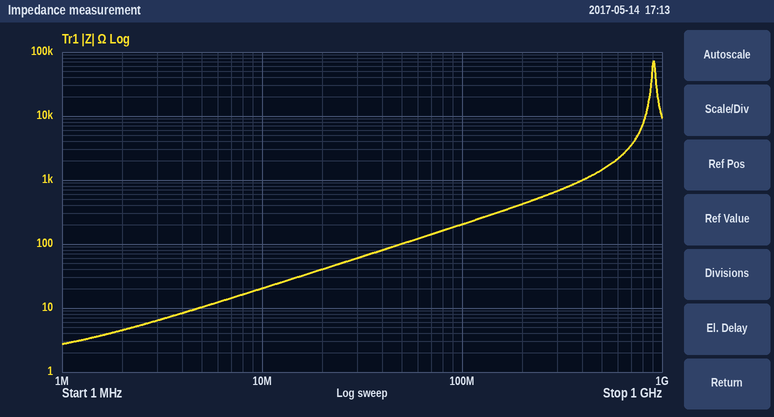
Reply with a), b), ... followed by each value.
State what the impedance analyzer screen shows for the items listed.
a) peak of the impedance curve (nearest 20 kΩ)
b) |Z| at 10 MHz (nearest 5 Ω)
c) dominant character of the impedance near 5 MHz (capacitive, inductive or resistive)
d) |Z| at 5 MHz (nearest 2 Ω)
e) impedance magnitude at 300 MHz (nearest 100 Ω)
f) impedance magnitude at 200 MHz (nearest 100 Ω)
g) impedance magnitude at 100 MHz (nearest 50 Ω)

a) 80 kΩ
b) 20 Ω
c) inductive
d) 10 Ω
e) 700 Ω
f) 400 Ω
g) 200 Ω
